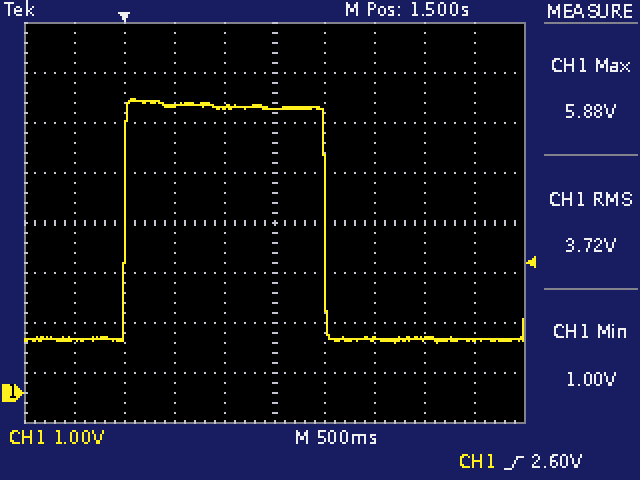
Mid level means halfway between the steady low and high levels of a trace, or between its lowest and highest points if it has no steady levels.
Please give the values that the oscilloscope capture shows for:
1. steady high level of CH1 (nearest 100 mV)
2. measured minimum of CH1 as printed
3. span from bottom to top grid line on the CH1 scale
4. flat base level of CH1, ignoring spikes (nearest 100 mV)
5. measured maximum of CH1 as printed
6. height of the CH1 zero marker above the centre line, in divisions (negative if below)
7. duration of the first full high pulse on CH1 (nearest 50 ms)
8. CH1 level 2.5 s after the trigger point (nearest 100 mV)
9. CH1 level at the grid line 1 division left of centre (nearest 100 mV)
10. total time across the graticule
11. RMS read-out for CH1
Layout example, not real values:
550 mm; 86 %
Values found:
5.7 V; 1.00 V; 8 V; 1.1 V; 5.88 V; -3.4 div; 2.00 s; 1.1 V; 5.7 V; 5 s; 3.72 V
